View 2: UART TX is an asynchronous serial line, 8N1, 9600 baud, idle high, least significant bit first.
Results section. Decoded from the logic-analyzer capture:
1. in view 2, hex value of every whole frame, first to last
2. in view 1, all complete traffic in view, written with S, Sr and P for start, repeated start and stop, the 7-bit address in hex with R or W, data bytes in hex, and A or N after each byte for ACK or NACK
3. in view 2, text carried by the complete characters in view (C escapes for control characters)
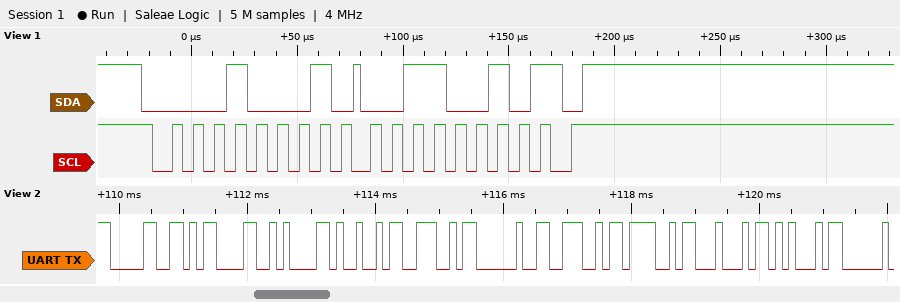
0x30 0x0D 0x0A 0x49 0x4E 0x20 0x4E 0x4F 0x44 0x45
S 08R A 32 N P
"0\r\nIN NODE"
